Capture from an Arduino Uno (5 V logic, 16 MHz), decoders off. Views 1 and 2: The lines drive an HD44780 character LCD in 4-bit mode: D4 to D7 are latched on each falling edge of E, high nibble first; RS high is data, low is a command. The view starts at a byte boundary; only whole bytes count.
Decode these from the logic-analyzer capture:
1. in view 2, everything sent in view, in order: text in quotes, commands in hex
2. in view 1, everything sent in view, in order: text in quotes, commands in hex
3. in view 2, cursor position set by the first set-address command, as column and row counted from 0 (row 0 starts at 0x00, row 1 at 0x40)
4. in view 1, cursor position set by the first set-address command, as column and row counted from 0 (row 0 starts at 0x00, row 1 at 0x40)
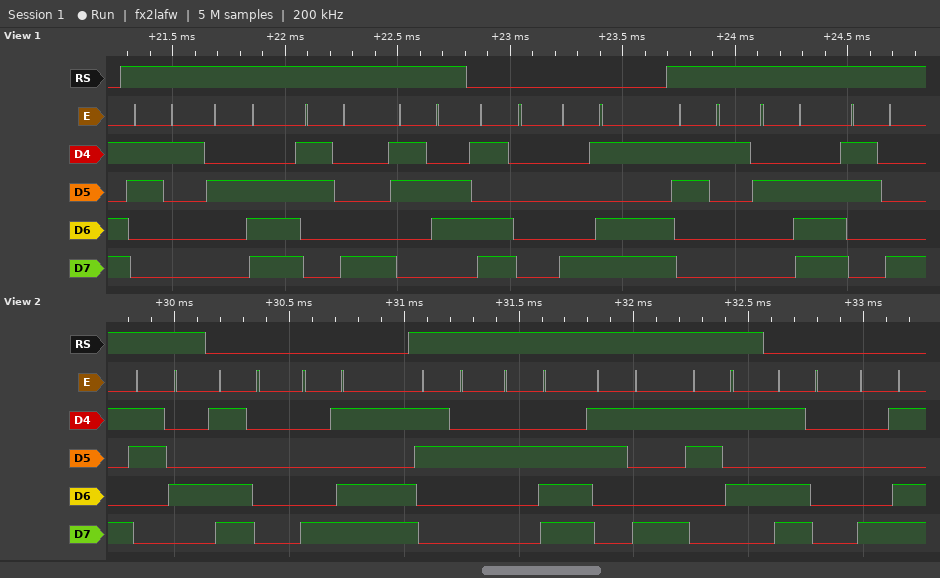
"4" 0xD0 0x8D "2.95" 0xD0 0x8D
"1.86" 0xD0 0x8D "1.8"
column 16, row 1
column 16, row 1
